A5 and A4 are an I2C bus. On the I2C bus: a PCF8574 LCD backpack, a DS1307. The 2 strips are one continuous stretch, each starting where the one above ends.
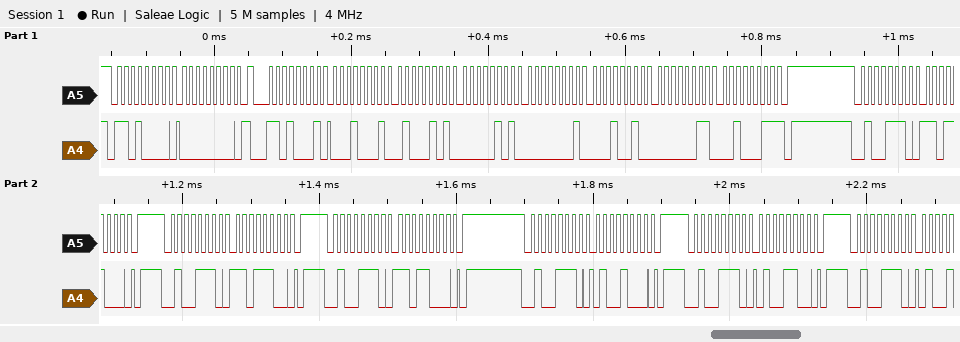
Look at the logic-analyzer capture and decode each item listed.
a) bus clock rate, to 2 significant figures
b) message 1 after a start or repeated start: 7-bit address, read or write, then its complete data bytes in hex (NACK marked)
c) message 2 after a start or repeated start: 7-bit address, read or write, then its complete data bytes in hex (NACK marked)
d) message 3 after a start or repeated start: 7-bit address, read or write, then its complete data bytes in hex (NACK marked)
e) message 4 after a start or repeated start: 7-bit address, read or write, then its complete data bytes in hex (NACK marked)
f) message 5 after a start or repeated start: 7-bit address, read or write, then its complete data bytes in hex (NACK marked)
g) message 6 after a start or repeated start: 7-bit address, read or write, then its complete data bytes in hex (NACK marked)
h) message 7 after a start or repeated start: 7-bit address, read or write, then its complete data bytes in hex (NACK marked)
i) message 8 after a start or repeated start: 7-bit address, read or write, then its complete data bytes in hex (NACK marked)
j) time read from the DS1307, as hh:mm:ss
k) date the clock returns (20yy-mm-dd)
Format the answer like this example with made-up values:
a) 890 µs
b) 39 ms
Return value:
a) 100 kHz
b) 0x68 write: 00
c) 0x68 read: 11 45 05 01 12 03 23 NACK
d) 0x27 write: D8
e) 0x27 write: DC
f) 0x27 write: D8
g) 0x27 write: 48
h) 0x27 write: 4C
i) 0x27 write
j) 05:45:11
k) 2023-03-12
